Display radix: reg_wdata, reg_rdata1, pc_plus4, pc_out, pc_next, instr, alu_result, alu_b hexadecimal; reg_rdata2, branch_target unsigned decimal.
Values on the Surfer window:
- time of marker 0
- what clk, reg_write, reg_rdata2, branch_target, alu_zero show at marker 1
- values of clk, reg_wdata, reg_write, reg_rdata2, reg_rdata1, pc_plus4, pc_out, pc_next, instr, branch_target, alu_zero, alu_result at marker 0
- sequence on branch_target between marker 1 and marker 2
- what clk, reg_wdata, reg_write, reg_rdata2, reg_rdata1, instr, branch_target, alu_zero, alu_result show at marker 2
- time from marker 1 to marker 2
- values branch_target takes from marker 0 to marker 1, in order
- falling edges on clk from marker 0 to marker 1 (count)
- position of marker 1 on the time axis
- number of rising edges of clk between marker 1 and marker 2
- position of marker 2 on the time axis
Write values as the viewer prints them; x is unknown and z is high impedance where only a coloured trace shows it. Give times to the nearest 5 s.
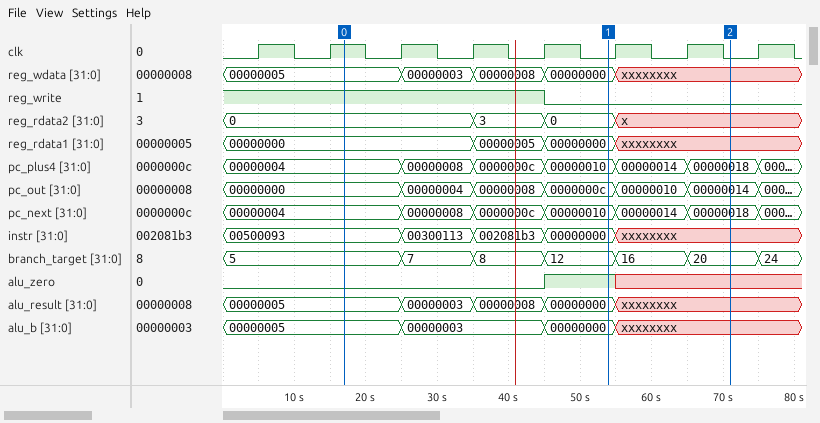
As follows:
15 s
clk=0, reg_write=0, reg_rdata2=0, branch_target=12, alu_zero=1
clk=1, reg_wdata=00000005, reg_write=1, reg_rdata2=0, reg_rdata1=00000000, pc_plus4=00000004, pc_out=00000000, pc_next=00000004, instr=00500093, branch_target=5, alu_zero=0, alu_result=00000005
12, 16, 20
clk=0, reg_wdata=xxxxxxxx, reg_write=0, reg_rdata2=x, reg_rdata1=xxxxxxxx, instr=xxxxxxxx, branch_target=20, alu_zero=x, alu_result=xxxxxxxx
15 s
5, 7, 8, 12
4
55 s
2
70 s
